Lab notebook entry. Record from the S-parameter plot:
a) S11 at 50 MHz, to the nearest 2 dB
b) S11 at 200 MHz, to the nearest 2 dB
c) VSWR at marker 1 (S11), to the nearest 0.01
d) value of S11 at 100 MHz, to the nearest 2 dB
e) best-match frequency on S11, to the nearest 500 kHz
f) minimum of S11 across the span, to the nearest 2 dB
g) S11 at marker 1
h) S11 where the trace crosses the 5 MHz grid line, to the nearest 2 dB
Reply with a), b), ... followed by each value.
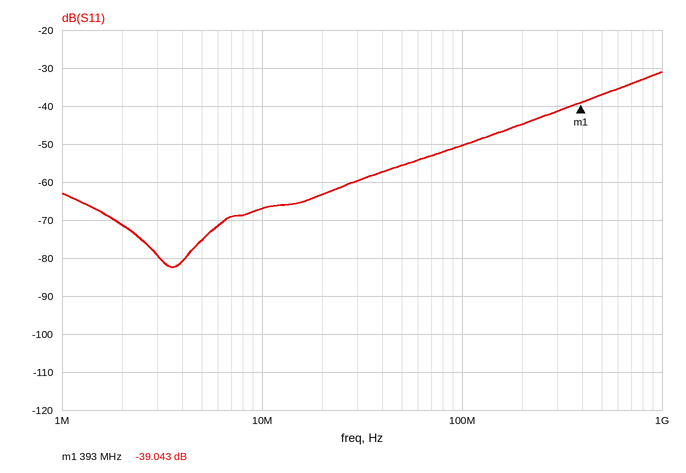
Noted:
a) -56 dB
b) -44 dB
c) 1.02
d) -50 dB
e) 3.5 MHz
f) -82 dB
g) -39.043 dB
h) -76 dB
